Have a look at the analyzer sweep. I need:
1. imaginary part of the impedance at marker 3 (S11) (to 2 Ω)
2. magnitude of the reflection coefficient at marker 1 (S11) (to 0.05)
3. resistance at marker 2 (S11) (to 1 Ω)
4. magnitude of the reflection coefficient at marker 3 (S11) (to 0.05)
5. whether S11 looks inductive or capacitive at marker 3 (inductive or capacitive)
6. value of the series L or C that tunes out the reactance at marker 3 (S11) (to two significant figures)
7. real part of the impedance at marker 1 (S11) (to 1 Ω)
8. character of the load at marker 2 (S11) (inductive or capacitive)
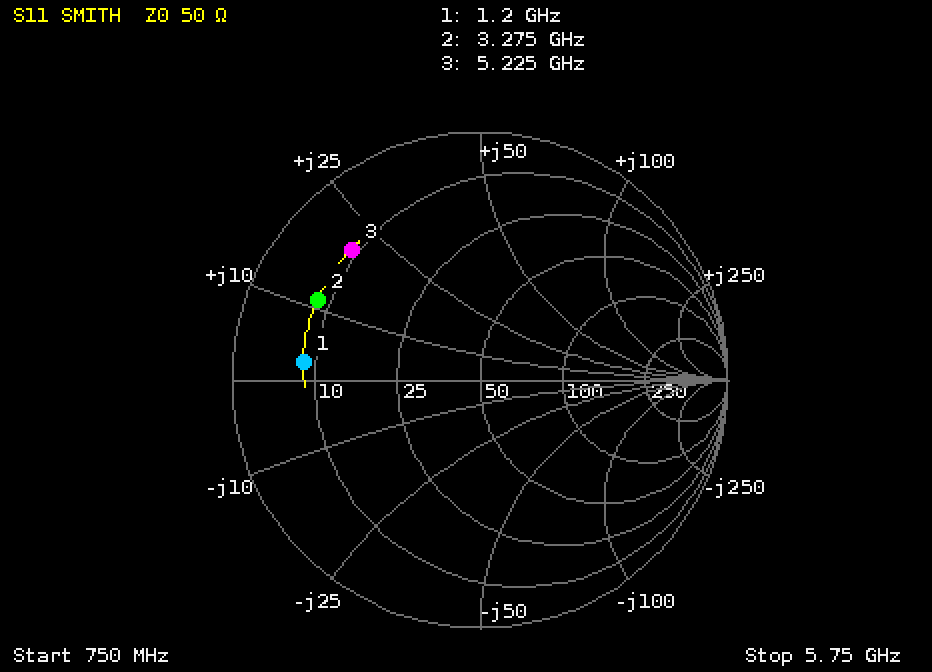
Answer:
+20 Ω
0.70
8 Ω
0.75
inductive
1.5 pF
8 Ω
inductive
